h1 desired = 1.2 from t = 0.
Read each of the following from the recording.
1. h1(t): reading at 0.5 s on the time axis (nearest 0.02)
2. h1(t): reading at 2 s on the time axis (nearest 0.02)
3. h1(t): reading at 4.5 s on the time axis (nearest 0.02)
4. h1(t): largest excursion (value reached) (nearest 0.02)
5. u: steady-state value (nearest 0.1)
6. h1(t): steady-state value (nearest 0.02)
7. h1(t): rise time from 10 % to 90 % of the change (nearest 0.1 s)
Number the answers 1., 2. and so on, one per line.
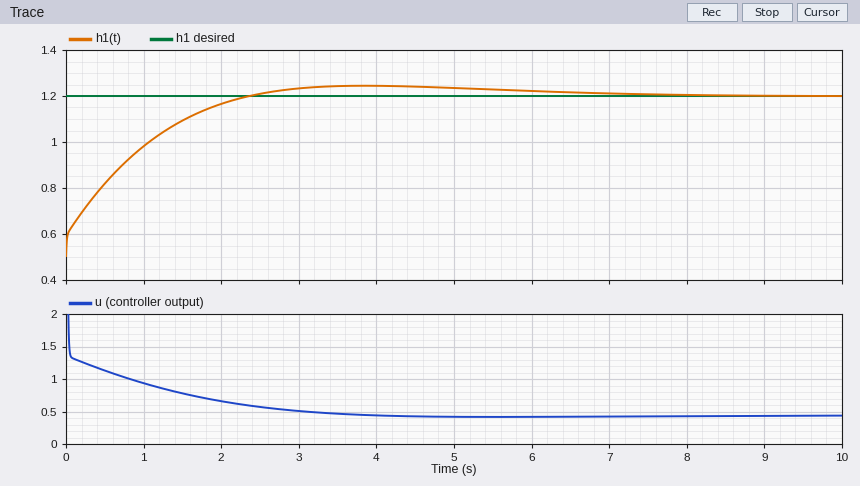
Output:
1. 0.82
2. 1.16
3. 1.24
4. 1.24
5. 0.4
6. 1.20
7. 1.7 s
